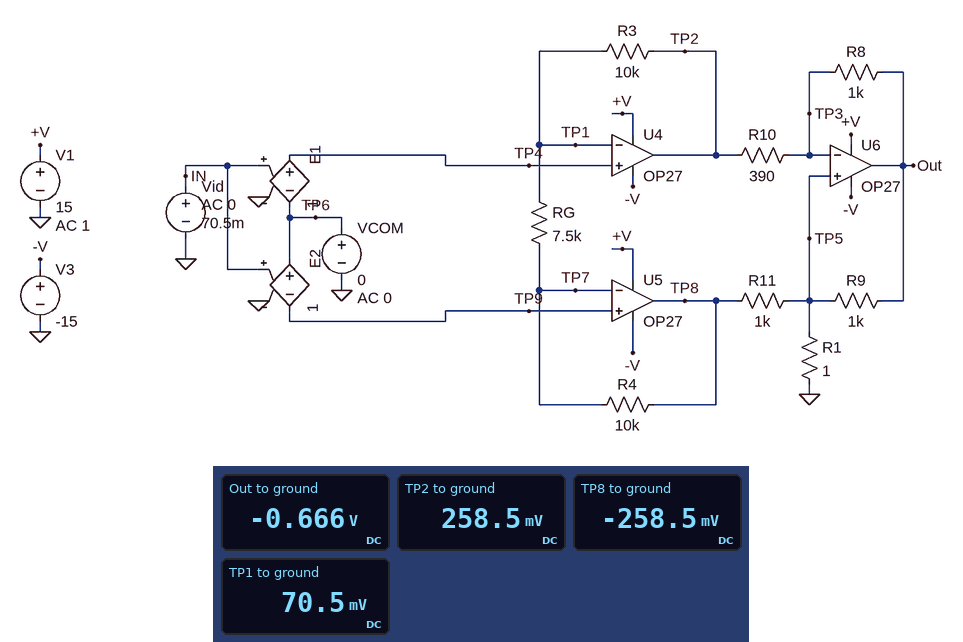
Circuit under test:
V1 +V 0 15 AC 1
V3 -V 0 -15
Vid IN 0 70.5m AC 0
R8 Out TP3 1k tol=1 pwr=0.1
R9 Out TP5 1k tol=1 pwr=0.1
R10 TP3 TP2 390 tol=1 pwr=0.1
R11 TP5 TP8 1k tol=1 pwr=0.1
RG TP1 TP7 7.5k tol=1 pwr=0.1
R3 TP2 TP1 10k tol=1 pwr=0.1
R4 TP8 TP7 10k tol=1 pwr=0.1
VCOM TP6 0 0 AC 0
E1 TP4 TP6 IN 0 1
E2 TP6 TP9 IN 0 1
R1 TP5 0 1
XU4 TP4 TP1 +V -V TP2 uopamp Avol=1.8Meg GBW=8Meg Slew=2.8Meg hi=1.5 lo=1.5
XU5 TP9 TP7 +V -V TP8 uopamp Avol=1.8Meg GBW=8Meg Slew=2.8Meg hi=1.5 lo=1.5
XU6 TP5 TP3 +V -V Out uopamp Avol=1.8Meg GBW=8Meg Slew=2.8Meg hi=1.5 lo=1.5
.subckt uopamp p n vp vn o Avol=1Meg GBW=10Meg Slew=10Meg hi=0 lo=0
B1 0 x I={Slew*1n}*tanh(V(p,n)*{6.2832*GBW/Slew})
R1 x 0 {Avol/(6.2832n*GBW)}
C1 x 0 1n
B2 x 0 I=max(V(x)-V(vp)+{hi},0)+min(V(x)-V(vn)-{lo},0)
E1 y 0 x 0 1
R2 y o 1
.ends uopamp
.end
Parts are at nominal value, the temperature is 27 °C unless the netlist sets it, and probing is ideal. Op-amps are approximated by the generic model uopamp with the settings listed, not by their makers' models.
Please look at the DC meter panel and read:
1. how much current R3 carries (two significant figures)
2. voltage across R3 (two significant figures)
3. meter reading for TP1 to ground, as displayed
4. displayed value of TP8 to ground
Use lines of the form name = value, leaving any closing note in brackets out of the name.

how much current R3 carries = 19 µA
voltage across R3 = 190 mV
meter reading for TP1 to ground, as displayed = 70.5 mV
displayed value of TP8 to ground = -258.5 mV
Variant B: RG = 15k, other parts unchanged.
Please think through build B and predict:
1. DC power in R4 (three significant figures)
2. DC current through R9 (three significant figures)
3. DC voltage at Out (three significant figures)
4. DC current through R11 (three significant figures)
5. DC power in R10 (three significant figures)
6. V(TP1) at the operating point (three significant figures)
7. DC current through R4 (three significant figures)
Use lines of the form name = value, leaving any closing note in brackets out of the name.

DC power in R4 = 884 nW
DC current through R9 = 423 µA
DC voltage at Out = -424 mV
DC current through R11 = 164 µA
DC power in R10 = 69.9 µW
V(TP1) at the operating point = 70.5 mV
DC current through R4 = 9.40 µA
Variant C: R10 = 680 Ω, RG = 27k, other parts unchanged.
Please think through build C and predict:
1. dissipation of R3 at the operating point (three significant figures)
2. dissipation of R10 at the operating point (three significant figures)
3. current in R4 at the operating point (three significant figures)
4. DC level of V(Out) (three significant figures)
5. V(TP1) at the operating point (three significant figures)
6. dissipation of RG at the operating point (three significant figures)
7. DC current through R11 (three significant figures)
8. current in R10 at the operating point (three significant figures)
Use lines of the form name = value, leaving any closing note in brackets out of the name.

dissipation of R3 at the operating point = 273 nW
dissipation of R10 at the operating point = 22.3 µW
current in R4 at the operating point = 5.22 µA
DC level of V(Out) = -181 mV
V(TP1) at the operating point = 70.5 mV
dissipation of RG at the operating point = 736 nW
DC current through R11 = 122 µA
current in R10 at the operating point = 181 µA
